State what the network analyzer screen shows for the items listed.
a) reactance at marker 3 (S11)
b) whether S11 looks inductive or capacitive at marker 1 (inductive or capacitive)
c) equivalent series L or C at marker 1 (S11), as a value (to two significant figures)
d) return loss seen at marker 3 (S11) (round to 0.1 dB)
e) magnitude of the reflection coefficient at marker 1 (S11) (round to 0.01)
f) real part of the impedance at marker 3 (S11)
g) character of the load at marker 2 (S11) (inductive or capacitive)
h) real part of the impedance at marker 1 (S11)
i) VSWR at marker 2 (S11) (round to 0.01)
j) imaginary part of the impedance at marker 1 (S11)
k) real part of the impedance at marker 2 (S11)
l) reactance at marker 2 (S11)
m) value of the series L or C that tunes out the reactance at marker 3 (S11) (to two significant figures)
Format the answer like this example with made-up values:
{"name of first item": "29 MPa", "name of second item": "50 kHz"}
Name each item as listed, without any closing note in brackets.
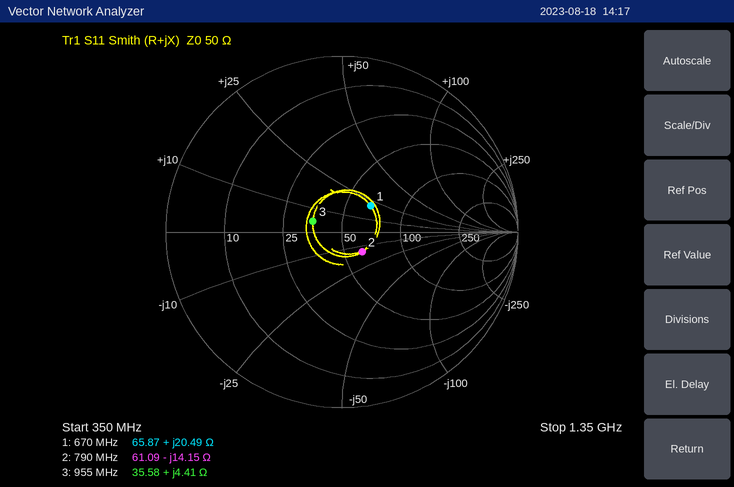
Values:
{"reactance at marker 3": "+4.41 Ω", "whether S11 looks inductive or capacitive at marker 1": "inductive", "equivalent series L or C at marker 1 (S11), as a value": "4.9 nH", "return loss seen at marker 3 (S11)": "15.1 dB", "magnitude of the reflection coefficient at marker 1 (S11)": "0.22", "real part of the impedance at marker 3": "35.58 Ω", "character of the load at marker 2 (S11)": "capacitive", "real part of the impedance at marker 1": "65.87 Ω", "VSWR at marker 2 (S11)": "1.38", "imaginary part of the impedance at marker 1": "+20.49 Ω", "real part of the impedance at marker 2": "61.09 Ω", "reactance at marker 2": "-14.15 Ω", "value of the series L or C that tunes out the reactance at marker 3 (S11)": "38 pF"}
